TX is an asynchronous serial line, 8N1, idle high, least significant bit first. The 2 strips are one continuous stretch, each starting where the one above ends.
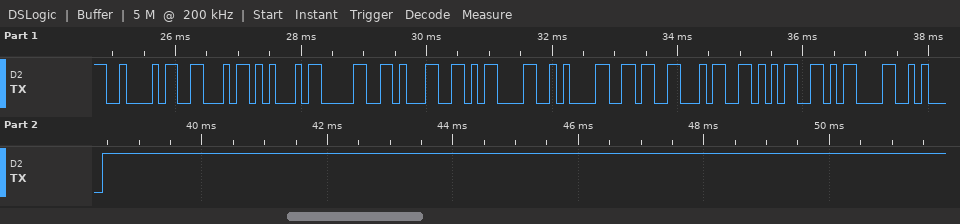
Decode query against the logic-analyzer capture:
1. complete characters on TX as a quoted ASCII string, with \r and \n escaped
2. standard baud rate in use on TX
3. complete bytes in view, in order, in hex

"BFE01\r\n645\r\n"
9600 baud
42 46 45 30 31 0D 0A 36 34 35 0D 0A
